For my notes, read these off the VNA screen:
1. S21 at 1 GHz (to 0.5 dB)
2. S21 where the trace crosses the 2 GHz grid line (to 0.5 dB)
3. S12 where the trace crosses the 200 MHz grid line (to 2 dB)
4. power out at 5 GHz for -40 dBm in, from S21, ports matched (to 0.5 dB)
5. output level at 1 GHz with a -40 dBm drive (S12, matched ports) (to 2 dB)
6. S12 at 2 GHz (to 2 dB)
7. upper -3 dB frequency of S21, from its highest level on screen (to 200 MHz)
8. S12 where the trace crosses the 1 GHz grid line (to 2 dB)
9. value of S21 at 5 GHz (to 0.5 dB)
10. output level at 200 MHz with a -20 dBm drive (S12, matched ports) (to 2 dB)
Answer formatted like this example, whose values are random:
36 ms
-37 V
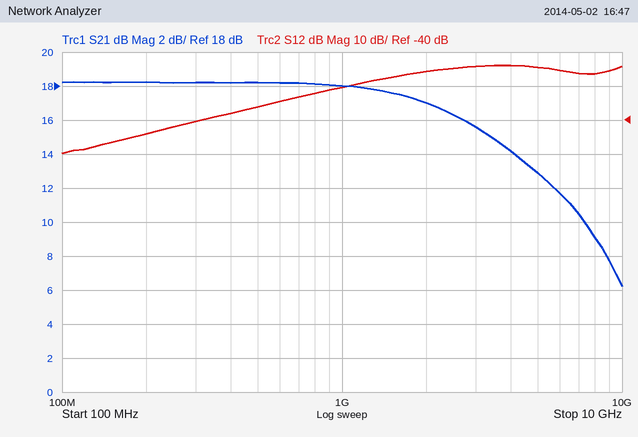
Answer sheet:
18.0 dB
17.0 dB
-44 dB
-27.0 dBm
-70 dBm
-26 dB
3.2 GHz
-30 dB
13.0 dB
-64 dBm
